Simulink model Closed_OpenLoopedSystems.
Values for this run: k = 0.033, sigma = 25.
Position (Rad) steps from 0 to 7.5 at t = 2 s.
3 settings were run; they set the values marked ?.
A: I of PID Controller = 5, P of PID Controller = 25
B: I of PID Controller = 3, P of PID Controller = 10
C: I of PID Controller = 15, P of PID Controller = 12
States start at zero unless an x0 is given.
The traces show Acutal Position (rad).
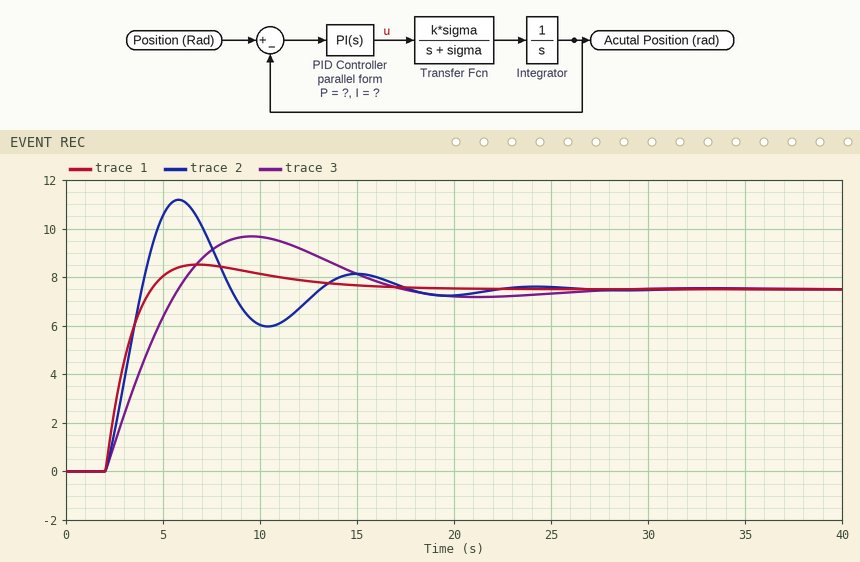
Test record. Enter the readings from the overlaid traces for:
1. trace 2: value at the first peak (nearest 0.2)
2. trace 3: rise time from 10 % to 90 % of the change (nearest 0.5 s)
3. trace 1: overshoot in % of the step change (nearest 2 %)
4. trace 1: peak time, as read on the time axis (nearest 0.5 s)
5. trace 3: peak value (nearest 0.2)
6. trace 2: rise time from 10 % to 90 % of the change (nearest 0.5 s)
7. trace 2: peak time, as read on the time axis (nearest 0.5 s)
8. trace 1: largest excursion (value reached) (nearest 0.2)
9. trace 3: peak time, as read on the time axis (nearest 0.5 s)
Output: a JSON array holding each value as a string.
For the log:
["11.2", "3.0 s", "14 %", "7.0 s", "9.6", "1.5 s", "6.0 s", "8.6", "9.5 s"]
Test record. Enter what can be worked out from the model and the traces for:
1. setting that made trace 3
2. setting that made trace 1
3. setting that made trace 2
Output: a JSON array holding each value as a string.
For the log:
["B", "A", "C"]
